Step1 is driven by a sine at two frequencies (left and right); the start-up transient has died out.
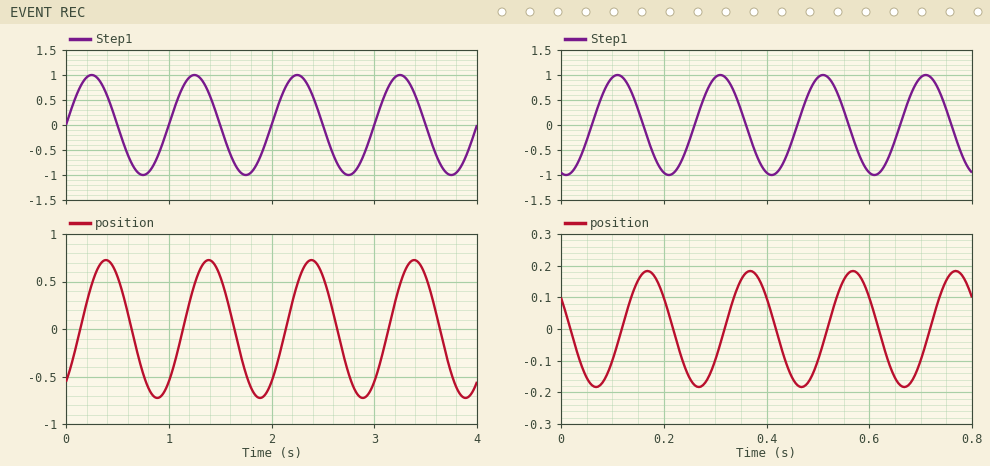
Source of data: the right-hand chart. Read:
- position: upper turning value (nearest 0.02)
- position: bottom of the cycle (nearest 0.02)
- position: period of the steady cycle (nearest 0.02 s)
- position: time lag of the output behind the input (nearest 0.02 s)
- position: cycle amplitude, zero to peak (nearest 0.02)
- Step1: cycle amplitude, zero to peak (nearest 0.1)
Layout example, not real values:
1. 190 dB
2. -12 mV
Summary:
1. 0.18
2. -0.18
3. 0.20 s
4. 0.06 s
5. 0.18
6. 1.0
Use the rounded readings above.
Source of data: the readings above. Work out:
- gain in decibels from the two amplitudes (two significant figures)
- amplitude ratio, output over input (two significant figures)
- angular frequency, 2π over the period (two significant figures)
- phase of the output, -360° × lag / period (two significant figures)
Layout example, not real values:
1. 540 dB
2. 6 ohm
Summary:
1. -15 dB
2. 0.18
3. 31 rad/s
4. -110°
